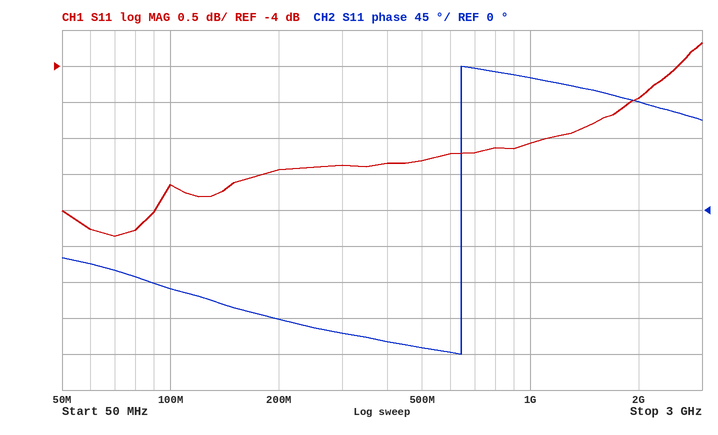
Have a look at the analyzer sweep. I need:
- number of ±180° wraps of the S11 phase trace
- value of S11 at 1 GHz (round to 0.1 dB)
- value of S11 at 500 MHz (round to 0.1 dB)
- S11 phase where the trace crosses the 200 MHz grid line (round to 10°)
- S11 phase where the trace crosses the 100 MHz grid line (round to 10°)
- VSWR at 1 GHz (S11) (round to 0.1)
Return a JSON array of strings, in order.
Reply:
["1", "-5.1 dB", "-5.3 dB", "-140°", "-100°", "3.5"]
